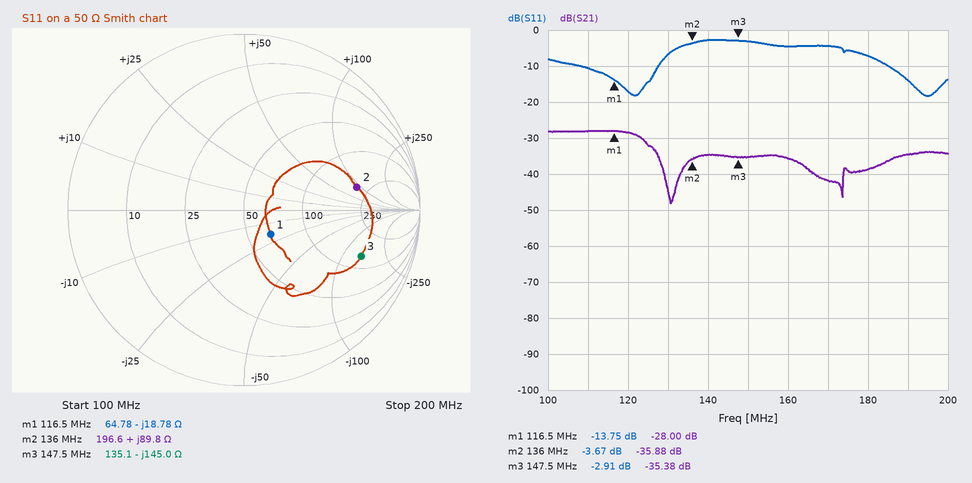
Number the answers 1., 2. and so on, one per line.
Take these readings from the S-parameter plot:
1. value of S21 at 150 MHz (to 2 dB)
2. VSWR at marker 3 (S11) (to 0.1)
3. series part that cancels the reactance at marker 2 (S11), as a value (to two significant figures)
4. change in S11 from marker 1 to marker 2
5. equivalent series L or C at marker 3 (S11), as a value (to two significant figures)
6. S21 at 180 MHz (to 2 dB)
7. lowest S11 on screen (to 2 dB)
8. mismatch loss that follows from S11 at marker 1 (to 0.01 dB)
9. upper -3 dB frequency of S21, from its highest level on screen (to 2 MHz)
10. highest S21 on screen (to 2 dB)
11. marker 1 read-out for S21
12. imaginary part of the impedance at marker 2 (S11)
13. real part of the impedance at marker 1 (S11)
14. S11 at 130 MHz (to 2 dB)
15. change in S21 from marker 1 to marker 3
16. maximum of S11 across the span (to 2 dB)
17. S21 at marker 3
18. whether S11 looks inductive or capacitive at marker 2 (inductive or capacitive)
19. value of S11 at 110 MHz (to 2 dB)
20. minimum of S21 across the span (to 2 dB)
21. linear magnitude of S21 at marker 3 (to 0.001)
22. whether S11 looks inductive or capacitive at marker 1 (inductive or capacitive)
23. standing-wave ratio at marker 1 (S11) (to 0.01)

1. -36 dB
2. 6.0
3. 13 pF
4. 10.08 dB
5. 7.4 pF
6. -38 dB
7. -18 dB
8. 0.19 dB
9. 124 MHz
10. -28 dB
11. -28.00 dB
12. +89.8 Ω
13. 64.78 Ω
14. -6 dB
15. -7.38 dB
16. -2 dB
17. -35.38 dB
18. inductive
19. -10 dB
20. -48 dB
21. 0.017
22. capacitive
23. 1.52
